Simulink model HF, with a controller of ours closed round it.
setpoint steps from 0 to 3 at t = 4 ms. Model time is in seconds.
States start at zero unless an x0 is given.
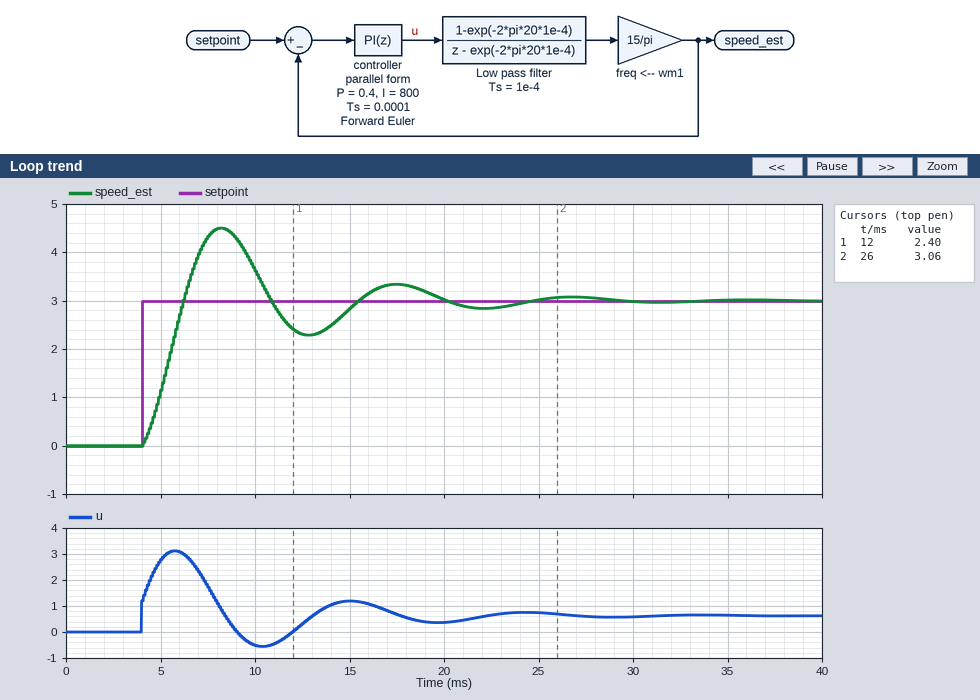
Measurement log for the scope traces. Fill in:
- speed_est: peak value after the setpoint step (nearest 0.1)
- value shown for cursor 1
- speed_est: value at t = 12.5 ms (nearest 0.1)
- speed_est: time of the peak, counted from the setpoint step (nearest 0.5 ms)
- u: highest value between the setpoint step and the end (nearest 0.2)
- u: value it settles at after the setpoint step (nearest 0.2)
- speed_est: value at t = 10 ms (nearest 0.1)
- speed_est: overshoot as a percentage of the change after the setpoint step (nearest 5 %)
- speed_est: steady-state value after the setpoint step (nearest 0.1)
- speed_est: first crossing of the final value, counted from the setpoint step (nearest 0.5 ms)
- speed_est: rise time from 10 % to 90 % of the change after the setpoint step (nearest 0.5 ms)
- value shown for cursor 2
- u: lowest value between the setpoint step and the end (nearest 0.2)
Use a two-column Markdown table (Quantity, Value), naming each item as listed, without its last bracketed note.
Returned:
| Quantity | Value |
|---|---|
| speed_est: peak value after the setpoint step | 4.5 |
| value shown for cursor 1 | 2.40 |
| speed_est: value at t = 12.5 ms | 2.3 |
| speed_est: time of the peak, counted from the setpoint step | 4.0 ms |
| u: highest value between the setpoint step and the end | 3.2 |
| u: value it settles at after the setpoint step | 0.6 |
| speed_est: value at t = 10 ms | 3.6 |
| speed_est: overshoot as a percentage of the change after the setpoint step | 50 % |
| speed_est: steady-state value after the setpoint step | 3.0 |
| speed_est: first crossing of the final value, counted from the setpoint step | 2.0 ms |
| speed_est: rise time from 10 % to 90 % of the change after the setpoint step | 1.5 ms |
| value shown for cursor 2 | 3.06 |
| u: lowest value between the setpoint step and the end | -0.6 |
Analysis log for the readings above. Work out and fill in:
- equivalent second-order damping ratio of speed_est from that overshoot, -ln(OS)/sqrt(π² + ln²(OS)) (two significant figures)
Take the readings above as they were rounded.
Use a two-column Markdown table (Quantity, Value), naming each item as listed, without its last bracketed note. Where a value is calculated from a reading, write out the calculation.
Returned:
| Quantity | Value |
|---|---|
| equivalent second-order damping ratio of speed_est from that overshoot, -ln(OS)/sqrt(π² + ln²(OS)) | ln(0.5) = -0.693; 0.693 / sqrt(9.870 + 0.480) = 0.22 |
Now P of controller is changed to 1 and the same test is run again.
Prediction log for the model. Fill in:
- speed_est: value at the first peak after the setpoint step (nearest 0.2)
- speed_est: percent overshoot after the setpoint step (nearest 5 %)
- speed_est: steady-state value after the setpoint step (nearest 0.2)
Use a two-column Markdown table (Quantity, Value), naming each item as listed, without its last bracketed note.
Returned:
| Quantity | Value |
|---|---|
| speed_est: value at the first peak after the setpoint step | 3.8 |
| speed_est: percent overshoot after the setpoint step | 25 % |
| speed_est: steady-state value after the setpoint step | 3.0 |
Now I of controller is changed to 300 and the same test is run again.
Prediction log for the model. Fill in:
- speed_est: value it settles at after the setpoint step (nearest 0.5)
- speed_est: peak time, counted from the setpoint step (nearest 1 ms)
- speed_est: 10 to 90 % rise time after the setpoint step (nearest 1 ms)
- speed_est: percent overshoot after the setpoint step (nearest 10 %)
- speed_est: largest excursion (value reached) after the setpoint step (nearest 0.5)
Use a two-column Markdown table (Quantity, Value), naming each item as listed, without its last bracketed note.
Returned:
| Quantity | Value |
|---|---|
| speed_est: value it settles at after the setpoint step | 3.0 |
| speed_est: peak time, counted from the setpoint step | 7 ms |
| speed_est: 10 to 90 % rise time after the setpoint step | 3 ms |
| speed_est: percent overshoot after the setpoint step | 30 % |
| speed_est: largest excursion (value reached) after the setpoint step | 4.0 |
